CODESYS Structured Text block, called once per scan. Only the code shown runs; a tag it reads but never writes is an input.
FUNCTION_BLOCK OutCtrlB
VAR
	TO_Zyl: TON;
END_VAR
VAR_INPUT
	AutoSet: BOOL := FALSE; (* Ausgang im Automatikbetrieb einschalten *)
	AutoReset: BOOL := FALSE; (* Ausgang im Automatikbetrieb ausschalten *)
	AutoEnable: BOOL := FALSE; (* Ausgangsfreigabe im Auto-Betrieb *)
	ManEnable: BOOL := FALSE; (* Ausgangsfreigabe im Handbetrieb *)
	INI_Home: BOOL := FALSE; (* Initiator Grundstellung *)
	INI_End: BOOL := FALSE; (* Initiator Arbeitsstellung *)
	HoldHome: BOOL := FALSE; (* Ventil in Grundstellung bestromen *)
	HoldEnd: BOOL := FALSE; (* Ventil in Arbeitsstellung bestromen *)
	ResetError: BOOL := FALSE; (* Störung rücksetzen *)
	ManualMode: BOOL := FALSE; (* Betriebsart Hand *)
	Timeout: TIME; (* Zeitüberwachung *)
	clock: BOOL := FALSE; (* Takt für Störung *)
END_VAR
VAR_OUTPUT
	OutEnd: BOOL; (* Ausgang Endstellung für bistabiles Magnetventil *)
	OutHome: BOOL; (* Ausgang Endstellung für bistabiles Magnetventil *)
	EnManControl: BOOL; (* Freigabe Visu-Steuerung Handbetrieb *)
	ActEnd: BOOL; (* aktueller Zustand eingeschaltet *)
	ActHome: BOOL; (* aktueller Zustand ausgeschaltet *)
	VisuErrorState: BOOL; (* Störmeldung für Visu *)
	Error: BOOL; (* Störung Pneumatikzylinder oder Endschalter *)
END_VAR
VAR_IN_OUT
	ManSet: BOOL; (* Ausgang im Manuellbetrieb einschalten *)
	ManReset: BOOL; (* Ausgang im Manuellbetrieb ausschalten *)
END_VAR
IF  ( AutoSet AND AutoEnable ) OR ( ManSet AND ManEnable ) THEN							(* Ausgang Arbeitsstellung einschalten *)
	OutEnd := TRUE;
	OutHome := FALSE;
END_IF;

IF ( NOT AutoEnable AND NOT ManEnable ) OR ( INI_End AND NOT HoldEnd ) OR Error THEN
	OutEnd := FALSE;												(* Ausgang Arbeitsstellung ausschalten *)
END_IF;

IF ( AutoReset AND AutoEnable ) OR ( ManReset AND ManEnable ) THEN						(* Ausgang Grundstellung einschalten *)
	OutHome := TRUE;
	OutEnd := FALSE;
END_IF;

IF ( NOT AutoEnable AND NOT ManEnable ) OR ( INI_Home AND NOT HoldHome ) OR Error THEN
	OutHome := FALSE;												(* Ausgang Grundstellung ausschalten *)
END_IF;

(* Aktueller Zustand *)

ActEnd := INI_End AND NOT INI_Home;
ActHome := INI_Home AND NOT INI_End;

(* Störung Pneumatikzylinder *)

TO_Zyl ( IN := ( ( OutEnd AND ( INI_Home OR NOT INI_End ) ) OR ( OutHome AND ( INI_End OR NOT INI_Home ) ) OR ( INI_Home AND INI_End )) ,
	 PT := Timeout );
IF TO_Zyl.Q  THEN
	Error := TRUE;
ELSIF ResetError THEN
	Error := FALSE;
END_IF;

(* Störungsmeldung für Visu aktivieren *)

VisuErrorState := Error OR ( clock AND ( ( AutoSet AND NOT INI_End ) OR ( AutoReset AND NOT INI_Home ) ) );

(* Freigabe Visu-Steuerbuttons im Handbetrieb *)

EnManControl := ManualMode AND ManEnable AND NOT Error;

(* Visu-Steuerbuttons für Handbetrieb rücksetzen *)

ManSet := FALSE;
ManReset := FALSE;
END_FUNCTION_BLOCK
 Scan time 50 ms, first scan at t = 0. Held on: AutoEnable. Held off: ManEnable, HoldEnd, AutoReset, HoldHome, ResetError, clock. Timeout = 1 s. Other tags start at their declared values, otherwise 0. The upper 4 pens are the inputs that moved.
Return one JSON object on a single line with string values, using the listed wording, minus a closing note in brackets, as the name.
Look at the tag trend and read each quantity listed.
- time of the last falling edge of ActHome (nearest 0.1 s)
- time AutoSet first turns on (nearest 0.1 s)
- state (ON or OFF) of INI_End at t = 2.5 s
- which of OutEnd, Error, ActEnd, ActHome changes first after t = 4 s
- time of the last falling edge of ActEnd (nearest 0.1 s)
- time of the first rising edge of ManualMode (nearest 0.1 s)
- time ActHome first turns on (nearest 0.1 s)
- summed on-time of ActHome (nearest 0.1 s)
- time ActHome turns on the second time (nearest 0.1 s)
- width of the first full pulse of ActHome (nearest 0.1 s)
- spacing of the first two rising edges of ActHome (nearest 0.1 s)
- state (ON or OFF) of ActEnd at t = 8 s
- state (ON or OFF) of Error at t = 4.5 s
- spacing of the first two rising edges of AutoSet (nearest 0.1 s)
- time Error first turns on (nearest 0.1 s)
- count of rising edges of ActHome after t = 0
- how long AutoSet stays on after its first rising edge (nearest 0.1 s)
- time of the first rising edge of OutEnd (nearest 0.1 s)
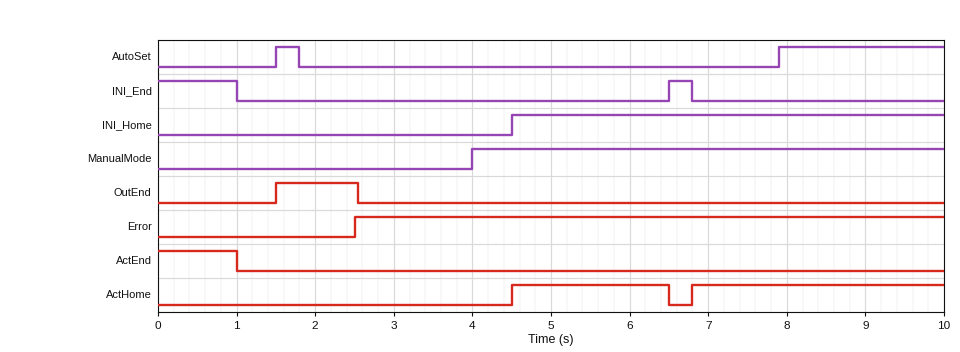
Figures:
{"time of the last falling edge of ActHome": "6.5 s", "time AutoSet first turns on": "1.5 s", "state (ON or OFF) of INI_End at t = 2.5 s": "OFF", "which of OutEnd, Error, ActEnd, ActHome changes first after t = 4 s": "ActHome", "time of the last falling edge of ActEnd": "1.0 s", "time of the first rising edge of ManualMode": "4.0 s", "time ActHome first turns on": "4.5 s", "summed on-time of ActHome": "5.2 s", "time ActHome turns on the second time": "6.8 s", "width of the first full pulse of ActHome": "2.0 s", "spacing of the first two rising edges of ActHome": "2.3 s", "state (ON or OFF) of ActEnd at t = 8 s": "OFF", "state (ON or OFF) of Error at t = 4.5 s": "ON", "spacing of the first two rising edges of AutoSet": "6.4 s", "time Error first turns on": "2.5 s", "count of rising edges of ActHome after t = 0": "2", "how long AutoSet stays on after its first rising edge": "0.3 s", "time of the first rising edge of OutEnd": "1.5 s"}
